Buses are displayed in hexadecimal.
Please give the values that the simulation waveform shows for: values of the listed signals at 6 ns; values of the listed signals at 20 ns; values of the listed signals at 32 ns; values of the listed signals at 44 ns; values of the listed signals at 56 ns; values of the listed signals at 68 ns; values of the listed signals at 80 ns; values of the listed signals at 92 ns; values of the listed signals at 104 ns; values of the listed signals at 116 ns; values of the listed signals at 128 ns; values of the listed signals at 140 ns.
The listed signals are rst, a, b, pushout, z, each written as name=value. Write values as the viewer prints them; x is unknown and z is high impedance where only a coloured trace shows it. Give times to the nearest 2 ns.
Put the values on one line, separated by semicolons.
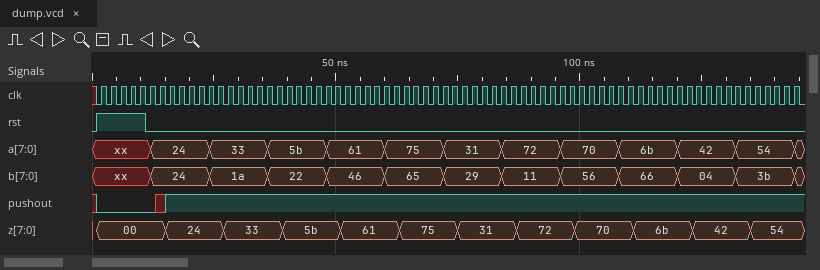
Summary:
rst=1, a=xx, b=xx, pushout=0, z=00; rst=0, a=24, b=24, pushout=1, z=24; rst=0, a=33, b=1a, pushout=1, z=33; rst=0, a=5b, b=22, pushout=1, z=5b; rst=0, a=61, b=46, pushout=1, z=61; rst=0, a=75, b=65, pushout=1, z=75; rst=0, a=31, b=29, pushout=1, z=31; rst=0, a=72, b=11, pushout=1, z=72; rst=0, a=70, b=56, pushout=1, z=70; rst=0, a=6b, b=66, pushout=1, z=6b; rst=0, a=42, b=04, pushout=1, z=42; rst=0, a=54, b=3b, pushout=1, z=54
